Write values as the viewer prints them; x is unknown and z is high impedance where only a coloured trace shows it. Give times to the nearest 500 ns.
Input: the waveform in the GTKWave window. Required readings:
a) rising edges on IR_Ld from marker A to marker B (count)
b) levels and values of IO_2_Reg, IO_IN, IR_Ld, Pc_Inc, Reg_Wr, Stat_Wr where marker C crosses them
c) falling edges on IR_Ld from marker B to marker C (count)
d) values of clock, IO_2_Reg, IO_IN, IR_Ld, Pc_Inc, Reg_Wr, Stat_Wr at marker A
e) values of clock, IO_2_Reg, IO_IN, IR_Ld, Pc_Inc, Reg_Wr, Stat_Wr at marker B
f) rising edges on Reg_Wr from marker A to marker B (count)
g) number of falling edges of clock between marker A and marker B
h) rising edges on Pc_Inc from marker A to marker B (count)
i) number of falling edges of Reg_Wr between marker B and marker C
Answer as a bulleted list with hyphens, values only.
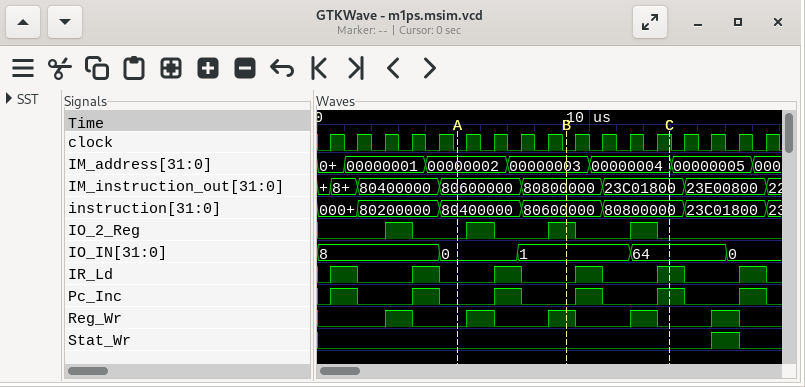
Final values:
- 1
- IO_2_Reg=0, IO_IN=64, IR_Ld=1, Pc_Inc=1, Reg_Wr=0, Stat_Wr=0
- 1
- clock=0, IO_2_Reg=0, IO_IN=0, IR_Ld=0, Pc_Inc=0, Reg_Wr=0, Stat_Wr=0
- clock=0, IO_2_Reg=1, IO_IN=1, IR_Ld=0, Pc_Inc=0, Reg_Wr=1, Stat_Wr=0
- 2
- 4
- 1
- 2
